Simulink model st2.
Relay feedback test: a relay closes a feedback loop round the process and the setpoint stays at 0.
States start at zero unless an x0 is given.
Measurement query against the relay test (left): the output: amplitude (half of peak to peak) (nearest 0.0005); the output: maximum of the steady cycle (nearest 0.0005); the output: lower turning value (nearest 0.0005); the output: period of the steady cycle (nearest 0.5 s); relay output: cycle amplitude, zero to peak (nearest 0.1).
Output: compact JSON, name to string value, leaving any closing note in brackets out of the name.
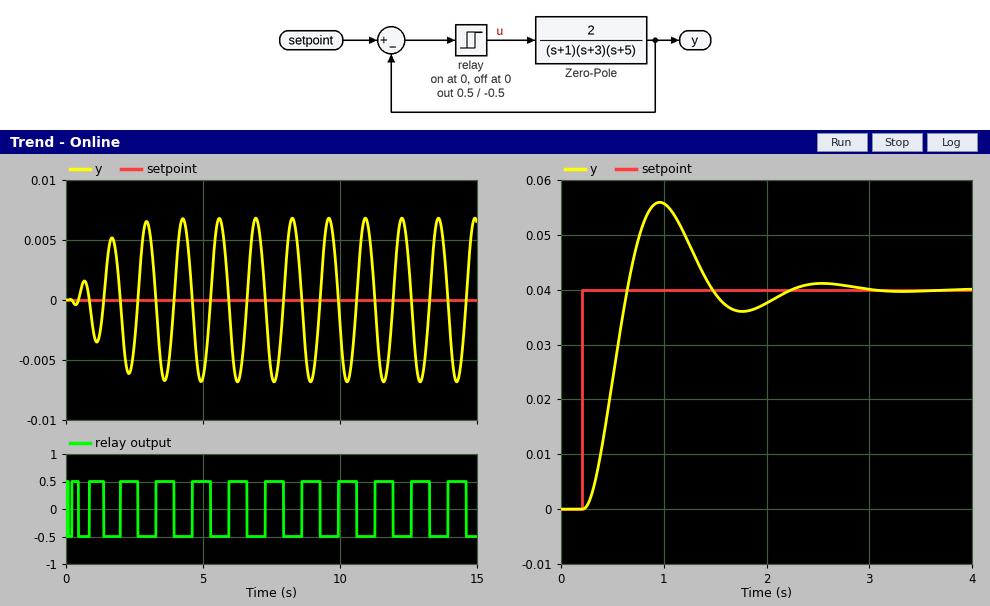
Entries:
{"the output: amplitude (half of peak to peak)": "0.0070", "the output: maximum of the steady cycle": "0.0070", "the output: lower turning value": "-0.0070", "the output: period of the steady cycle": "1.5 s", "relay output: cycle amplitude, zero to peak": "0.5"}
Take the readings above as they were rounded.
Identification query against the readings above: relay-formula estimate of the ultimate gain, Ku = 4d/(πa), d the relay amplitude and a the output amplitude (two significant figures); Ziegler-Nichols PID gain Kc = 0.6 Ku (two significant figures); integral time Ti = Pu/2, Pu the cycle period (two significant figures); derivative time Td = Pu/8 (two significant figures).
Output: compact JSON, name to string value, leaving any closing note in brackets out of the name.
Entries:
{"relay-formula estimate of the ultimate gain, Ku = 4d/(πa), d the relay amplitude and a the output amplitude": "91", "Ziegler-Nichols PID gain Kc = 0.6 Ku": "55", "integral time Ti = Pu/2, Pu the cycle period": "0.75 s", "derivative time Td = Pu/8": "0.19 s"}
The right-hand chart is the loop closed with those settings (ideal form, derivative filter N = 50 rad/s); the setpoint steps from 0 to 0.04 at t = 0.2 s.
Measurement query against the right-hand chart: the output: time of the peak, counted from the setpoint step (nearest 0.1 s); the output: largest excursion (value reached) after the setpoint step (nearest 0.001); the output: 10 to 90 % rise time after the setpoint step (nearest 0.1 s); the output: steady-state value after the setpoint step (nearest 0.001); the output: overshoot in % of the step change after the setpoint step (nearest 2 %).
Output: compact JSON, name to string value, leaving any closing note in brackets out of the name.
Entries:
{"the output: time of the peak, counted from the setpoint step": "0.8 s", "the output: largest excursion (value reached) after the setpoint step": "0.056", "the output: 10 to 90 % rise time after the setpoint step": "0.3 s", "the output: steady-state value after the setpoint step": "0.040", "the output: overshoot in % of the step change after the setpoint step": "40 %"}
